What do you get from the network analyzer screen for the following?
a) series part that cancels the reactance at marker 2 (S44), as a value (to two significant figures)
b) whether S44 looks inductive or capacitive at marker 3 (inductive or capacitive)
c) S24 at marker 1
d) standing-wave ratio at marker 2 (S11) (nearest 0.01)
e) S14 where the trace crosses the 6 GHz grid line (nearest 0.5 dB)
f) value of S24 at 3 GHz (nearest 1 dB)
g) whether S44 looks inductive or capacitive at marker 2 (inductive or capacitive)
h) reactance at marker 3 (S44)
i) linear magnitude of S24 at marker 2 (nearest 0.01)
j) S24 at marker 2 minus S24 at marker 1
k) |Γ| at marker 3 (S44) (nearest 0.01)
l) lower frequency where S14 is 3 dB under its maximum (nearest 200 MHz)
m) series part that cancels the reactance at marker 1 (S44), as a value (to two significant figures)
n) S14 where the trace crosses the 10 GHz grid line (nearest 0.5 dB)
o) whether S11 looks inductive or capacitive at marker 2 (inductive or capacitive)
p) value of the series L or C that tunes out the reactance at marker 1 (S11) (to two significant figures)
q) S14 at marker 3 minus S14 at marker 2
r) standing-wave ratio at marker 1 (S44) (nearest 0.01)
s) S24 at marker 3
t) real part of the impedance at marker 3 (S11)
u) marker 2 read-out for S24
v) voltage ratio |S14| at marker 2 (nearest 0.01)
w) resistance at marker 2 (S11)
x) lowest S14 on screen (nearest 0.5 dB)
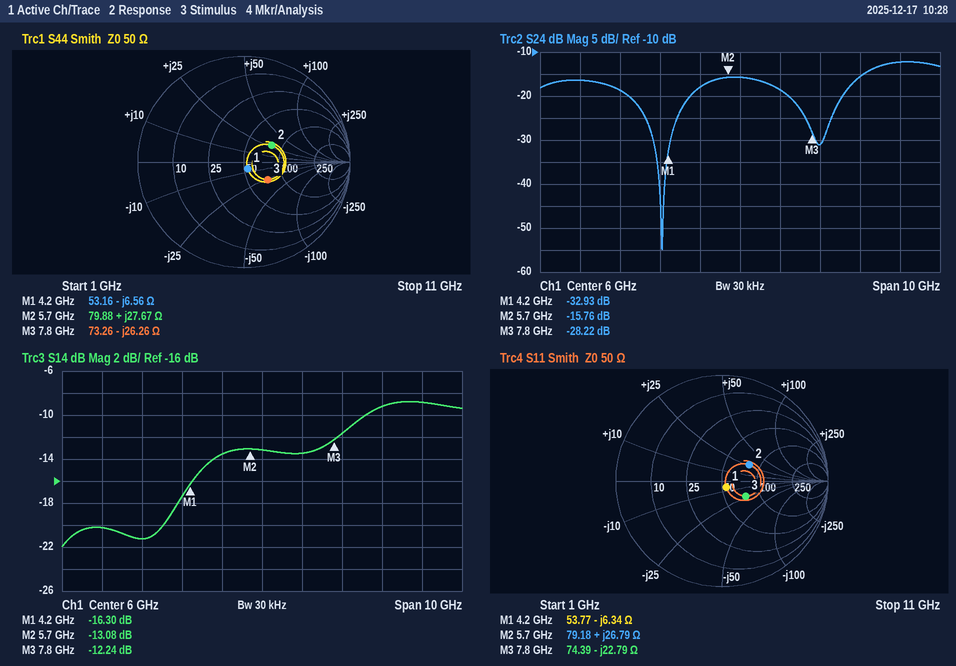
1.0 pF
capacitive
-32.93 dB
1.86
-13.0 dB
-19 dB
inductive
-26.26 Ω
0.16
17.17 dB
0.28
8.0 GHz
250 pH
-9.0 dB
inductive
240 pH
0.84 dB
1.15
-28.22 dB
74.39 Ω
-15.76 dB
0.22
79.18 Ω
-22.0 dB
